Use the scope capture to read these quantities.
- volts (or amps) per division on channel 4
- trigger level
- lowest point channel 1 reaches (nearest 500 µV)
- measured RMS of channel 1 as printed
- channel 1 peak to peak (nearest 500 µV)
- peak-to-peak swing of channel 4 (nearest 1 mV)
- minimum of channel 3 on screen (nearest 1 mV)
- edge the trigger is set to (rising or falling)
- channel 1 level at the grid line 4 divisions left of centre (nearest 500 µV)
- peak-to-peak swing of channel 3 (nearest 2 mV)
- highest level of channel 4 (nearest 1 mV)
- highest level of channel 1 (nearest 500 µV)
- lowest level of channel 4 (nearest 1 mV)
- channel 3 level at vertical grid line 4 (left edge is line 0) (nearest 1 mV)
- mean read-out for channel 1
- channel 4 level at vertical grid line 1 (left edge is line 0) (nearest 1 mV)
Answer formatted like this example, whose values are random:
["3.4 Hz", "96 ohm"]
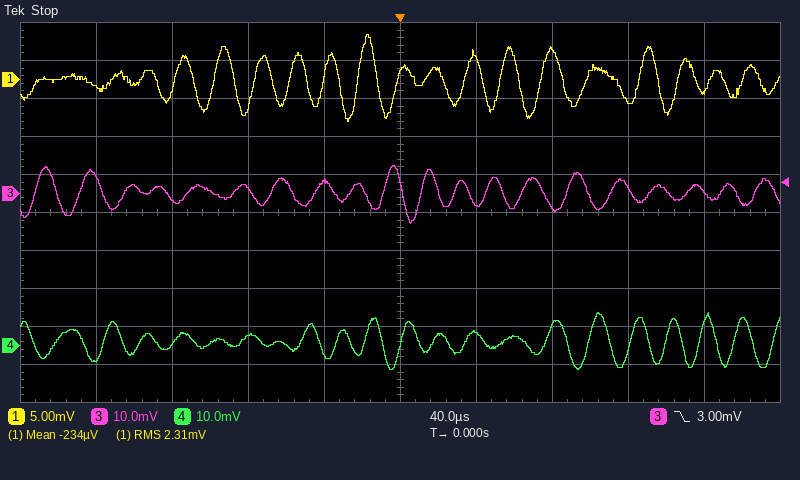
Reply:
["10 mV", "3.00 mV", "-5.5 mV", "2.31 mV", "11.5 mV", "15 mV", "-8 mV", "falling", "-1.0 mV", "16 mV", "9 mV", "6.0 mV", "-6 mV", "3 mV", "-234 µV", "-3 mV"]
